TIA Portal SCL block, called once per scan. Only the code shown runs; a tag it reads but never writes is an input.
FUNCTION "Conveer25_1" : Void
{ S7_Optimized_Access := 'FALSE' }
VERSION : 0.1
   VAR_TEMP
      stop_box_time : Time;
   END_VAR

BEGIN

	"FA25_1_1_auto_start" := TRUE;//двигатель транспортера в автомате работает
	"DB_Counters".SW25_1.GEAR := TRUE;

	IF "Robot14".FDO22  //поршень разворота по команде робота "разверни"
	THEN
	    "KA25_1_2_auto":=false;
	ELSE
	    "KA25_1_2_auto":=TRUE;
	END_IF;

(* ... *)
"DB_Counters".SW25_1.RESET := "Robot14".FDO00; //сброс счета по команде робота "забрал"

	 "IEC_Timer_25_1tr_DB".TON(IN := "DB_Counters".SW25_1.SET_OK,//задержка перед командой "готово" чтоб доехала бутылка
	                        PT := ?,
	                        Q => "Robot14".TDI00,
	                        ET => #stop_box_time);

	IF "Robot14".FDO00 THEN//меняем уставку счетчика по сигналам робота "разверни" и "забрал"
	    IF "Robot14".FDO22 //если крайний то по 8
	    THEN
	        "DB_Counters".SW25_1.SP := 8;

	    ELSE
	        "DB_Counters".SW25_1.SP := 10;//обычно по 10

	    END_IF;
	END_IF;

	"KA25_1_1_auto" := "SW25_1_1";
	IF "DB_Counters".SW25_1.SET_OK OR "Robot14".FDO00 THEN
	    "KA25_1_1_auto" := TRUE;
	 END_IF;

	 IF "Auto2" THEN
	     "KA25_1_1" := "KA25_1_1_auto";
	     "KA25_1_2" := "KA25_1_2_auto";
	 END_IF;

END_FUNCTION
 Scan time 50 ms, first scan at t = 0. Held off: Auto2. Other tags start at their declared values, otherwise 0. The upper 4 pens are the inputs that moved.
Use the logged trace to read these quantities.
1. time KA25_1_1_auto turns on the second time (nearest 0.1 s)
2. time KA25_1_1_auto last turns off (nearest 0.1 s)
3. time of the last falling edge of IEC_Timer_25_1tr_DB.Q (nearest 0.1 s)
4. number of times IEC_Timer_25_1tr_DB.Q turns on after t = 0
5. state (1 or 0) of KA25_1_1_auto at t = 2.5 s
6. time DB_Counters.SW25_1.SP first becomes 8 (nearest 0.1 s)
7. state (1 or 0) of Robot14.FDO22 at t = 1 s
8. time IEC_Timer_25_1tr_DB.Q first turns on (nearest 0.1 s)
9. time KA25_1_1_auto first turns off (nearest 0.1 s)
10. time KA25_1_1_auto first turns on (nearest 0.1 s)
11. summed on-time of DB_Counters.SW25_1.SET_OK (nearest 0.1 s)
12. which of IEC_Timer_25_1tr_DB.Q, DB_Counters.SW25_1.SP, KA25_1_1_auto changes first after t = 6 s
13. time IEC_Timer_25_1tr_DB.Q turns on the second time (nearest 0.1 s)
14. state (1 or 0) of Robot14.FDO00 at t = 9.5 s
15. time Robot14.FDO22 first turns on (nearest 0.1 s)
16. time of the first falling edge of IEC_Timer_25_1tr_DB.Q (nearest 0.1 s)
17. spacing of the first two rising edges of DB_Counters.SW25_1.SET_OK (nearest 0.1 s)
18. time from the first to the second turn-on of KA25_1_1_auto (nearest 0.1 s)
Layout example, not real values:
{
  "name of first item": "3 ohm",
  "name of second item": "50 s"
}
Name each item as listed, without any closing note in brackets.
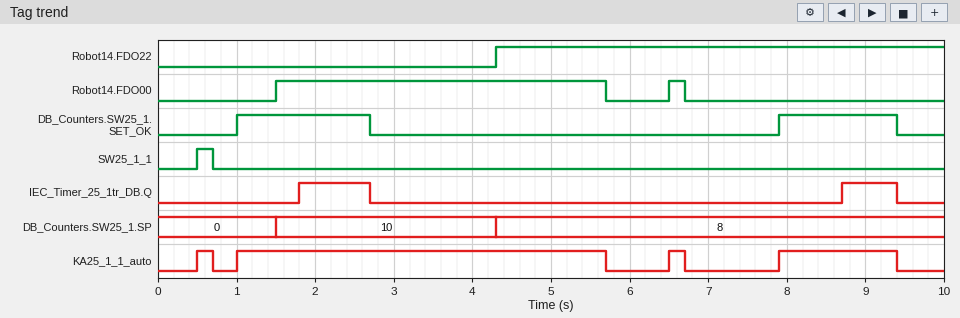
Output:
{
  "time KA25_1_1_auto turns on the second time": "1.0 s",
  "time KA25_1_1_auto last turns off": "9.4 s",
  "time of the last falling edge of IEC_Timer_25_1tr_DB.Q": "9.4 s",
  "number of times IEC_Timer_25_1tr_DB.Q turns on after t = 0": "2",
  "state (1 or 0) of KA25_1_1_auto at t = 2.5 s": "1",
  "time DB_Counters.SW25_1.SP first becomes 8": "4.3 s",
  "state (1 or 0) of Robot14.FDO22 at t = 1 s": "0",
  "time IEC_Timer_25_1tr_DB.Q first turns on": "1.8 s",
  "time KA25_1_1_auto first turns off": "0.7 s",
  "time KA25_1_1_auto first turns on": "0.5 s",
  "summed on-time of DB_Counters.SW25_1.SET_OK": "3.2 s",
  "which of IEC_Timer_25_1tr_DB.Q, DB_Counters.SW25_1.SP, KA25_1_1_auto changes first after t = 6 s": "KA25_1_1_auto",
  "time IEC_Timer_25_1tr_DB.Q turns on the second time": "8.7 s",
  "state (1 or 0) of Robot14.FDO00 at t = 9.5 s": "0",
  "time Robot14.FDO22 first turns on": "4.3 s",
  "time of the first falling edge of IEC_Timer_25_1tr_DB.Q": "2.7 s",
  "spacing of the first two rising edges of DB_Counters.SW25_1.SET_OK": "6.9 s",
  "time from the first to the second turn-on of KA25_1_1_auto": "0.5 s"
}
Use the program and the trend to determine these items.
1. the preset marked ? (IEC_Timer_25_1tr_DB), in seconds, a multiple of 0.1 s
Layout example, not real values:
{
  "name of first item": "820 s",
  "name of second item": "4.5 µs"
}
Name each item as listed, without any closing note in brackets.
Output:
{
  "the preset marked ? (IEC_Timer_25_1tr_DB), in seconds, a multiple of 0.1 s": "0.8 s"
}
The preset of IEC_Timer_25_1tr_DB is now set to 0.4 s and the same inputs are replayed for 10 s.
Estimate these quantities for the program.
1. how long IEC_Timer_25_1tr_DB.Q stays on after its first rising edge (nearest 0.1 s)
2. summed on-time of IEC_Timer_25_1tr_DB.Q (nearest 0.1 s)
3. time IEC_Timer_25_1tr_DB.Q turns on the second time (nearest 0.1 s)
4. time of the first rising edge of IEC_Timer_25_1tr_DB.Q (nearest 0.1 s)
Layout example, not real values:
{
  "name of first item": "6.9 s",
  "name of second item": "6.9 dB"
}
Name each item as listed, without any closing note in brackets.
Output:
{
  "how long IEC_Timer_25_1tr_DB.Q stays on after its first rising edge": "1.3 s",
  "summed on-time of IEC_Timer_25_1tr_DB.Q": "2.4 s",
  "time IEC_Timer_25_1tr_DB.Q turns on the second time": "8.3 s",
  "time of the first rising edge of IEC_Timer_25_1tr_DB.Q": "1.4 s"
}
